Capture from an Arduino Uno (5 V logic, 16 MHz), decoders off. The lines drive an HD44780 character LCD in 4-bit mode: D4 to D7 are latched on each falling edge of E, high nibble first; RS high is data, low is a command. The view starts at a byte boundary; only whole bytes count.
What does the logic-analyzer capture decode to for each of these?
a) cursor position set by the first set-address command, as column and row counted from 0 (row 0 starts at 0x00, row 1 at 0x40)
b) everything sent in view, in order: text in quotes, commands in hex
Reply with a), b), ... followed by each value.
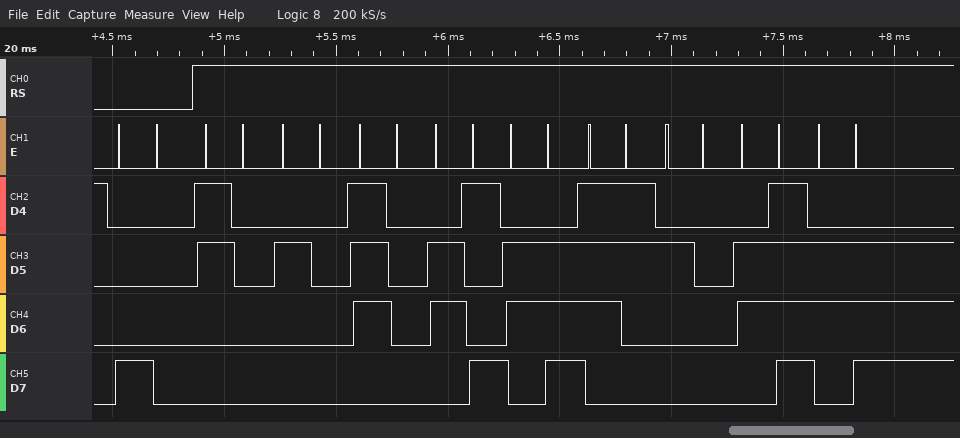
a) column 0, row 0
b) 0x80 "0 pins on"
